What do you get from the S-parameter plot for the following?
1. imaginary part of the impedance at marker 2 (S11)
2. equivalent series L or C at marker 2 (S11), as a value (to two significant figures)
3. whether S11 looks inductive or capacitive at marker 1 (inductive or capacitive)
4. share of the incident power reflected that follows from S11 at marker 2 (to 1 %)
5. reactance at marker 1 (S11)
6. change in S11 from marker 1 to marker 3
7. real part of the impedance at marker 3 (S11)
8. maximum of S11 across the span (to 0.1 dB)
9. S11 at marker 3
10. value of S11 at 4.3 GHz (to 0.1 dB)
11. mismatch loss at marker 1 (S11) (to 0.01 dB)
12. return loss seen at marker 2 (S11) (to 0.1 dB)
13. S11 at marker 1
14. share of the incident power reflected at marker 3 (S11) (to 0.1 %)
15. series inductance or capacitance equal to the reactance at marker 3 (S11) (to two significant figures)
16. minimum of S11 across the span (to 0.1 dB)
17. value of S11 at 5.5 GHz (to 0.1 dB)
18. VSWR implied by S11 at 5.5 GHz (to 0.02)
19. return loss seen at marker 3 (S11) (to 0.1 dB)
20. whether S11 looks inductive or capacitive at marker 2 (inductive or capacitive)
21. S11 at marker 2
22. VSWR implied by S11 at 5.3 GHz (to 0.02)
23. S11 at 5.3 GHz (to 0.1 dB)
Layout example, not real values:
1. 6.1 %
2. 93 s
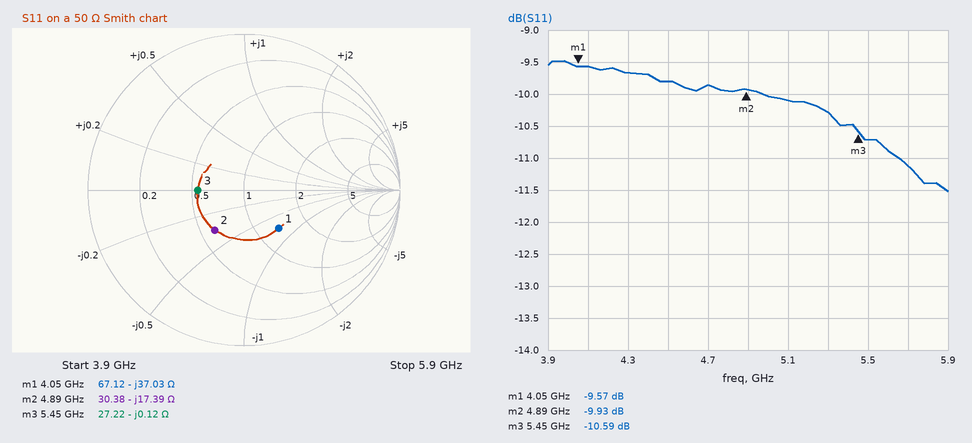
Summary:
1. -17.39 Ω
2. 1.9 pF
3. capacitive
4. 10 %
5. -37.03 Ω
6. -1.02 dB
7. 27.22 Ω
8. -9.5 dB
9. -10.59 dB
10. -9.7 dB
11. 0.51 dB
12. 9.9 dB
13. -9.57 dB
14. 8.7 %
15. 240 pF
16. -11.5 dB
17. -10.7 dB
18. 1.82
19. 10.6 dB
20. capacitive
21. -9.93 dB
22. 1.88
23. -10.3 dB
